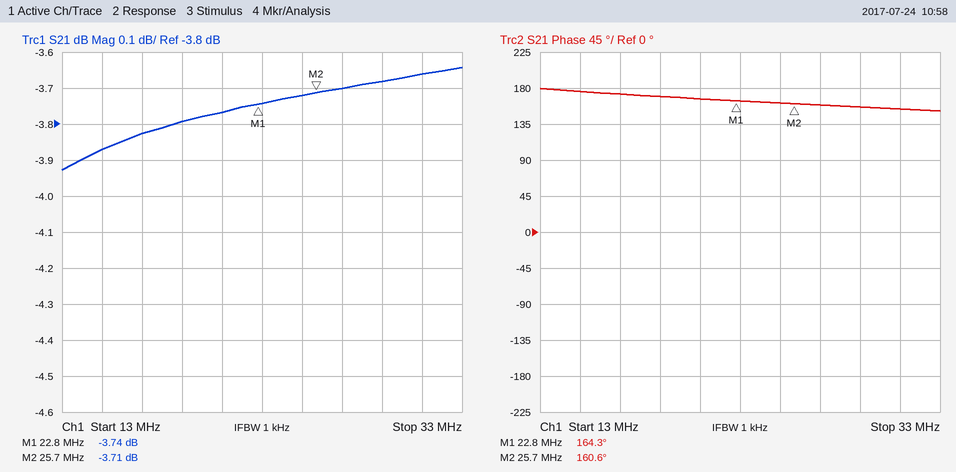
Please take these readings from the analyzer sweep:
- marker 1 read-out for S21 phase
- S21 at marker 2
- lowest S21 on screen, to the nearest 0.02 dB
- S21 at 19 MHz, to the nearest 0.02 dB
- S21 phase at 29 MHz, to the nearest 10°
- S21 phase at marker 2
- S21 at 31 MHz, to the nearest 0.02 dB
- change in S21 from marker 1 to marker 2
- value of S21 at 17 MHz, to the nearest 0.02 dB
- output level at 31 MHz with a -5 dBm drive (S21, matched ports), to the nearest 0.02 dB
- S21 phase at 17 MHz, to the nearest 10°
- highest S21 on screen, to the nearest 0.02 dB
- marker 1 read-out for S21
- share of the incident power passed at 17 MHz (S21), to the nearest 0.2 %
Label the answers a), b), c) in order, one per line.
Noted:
a) 164.3°
b) -3.71 dB
c) -3.92 dB
d) -3.80 dB
e) 160°
f) 160.6°
g) -3.66 dB
h) 0.03 dB
i) -3.82 dB
j) -8.66 dBm
k) 170°
l) -3.64 dB
m) -3.74 dB
n) 41.4 %
